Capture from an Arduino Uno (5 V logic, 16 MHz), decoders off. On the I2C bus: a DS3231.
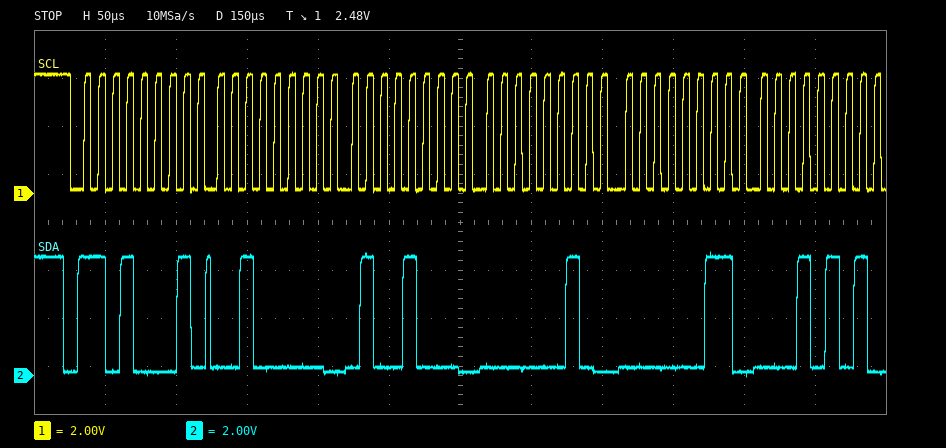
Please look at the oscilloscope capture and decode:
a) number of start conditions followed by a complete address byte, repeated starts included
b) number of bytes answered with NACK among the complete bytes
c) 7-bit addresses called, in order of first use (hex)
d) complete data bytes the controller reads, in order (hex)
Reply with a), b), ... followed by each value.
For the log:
a) 1
b) 0
c) 0x68
d) 20 48 02 03 15
